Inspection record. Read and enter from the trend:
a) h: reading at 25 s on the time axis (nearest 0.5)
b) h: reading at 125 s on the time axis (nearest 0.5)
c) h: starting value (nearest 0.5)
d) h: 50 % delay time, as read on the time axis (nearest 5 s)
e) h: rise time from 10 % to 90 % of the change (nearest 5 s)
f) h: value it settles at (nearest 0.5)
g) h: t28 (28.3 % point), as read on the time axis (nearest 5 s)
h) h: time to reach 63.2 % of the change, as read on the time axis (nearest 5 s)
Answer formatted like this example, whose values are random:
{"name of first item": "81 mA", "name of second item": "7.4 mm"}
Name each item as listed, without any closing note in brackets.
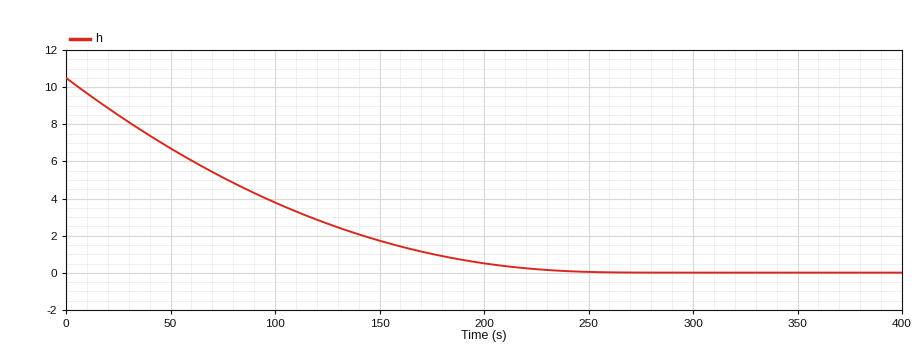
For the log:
{"h: reading at 25 s on the time axis": "8.5", "h: reading at 125 s on the time axis": "2.5", "h: starting value": "10.5", "h: 50 % delay time, as read on the time axis": "75 s", "h: rise time from 10 % to 90 % of the change": "160 s", "h: value it settles at": "0.0", "h: t28 (28.3 % point), as read on the time axis": "40 s", "h: time to reach 63.2 % of the change, as read on the time axis": "100 s"}
